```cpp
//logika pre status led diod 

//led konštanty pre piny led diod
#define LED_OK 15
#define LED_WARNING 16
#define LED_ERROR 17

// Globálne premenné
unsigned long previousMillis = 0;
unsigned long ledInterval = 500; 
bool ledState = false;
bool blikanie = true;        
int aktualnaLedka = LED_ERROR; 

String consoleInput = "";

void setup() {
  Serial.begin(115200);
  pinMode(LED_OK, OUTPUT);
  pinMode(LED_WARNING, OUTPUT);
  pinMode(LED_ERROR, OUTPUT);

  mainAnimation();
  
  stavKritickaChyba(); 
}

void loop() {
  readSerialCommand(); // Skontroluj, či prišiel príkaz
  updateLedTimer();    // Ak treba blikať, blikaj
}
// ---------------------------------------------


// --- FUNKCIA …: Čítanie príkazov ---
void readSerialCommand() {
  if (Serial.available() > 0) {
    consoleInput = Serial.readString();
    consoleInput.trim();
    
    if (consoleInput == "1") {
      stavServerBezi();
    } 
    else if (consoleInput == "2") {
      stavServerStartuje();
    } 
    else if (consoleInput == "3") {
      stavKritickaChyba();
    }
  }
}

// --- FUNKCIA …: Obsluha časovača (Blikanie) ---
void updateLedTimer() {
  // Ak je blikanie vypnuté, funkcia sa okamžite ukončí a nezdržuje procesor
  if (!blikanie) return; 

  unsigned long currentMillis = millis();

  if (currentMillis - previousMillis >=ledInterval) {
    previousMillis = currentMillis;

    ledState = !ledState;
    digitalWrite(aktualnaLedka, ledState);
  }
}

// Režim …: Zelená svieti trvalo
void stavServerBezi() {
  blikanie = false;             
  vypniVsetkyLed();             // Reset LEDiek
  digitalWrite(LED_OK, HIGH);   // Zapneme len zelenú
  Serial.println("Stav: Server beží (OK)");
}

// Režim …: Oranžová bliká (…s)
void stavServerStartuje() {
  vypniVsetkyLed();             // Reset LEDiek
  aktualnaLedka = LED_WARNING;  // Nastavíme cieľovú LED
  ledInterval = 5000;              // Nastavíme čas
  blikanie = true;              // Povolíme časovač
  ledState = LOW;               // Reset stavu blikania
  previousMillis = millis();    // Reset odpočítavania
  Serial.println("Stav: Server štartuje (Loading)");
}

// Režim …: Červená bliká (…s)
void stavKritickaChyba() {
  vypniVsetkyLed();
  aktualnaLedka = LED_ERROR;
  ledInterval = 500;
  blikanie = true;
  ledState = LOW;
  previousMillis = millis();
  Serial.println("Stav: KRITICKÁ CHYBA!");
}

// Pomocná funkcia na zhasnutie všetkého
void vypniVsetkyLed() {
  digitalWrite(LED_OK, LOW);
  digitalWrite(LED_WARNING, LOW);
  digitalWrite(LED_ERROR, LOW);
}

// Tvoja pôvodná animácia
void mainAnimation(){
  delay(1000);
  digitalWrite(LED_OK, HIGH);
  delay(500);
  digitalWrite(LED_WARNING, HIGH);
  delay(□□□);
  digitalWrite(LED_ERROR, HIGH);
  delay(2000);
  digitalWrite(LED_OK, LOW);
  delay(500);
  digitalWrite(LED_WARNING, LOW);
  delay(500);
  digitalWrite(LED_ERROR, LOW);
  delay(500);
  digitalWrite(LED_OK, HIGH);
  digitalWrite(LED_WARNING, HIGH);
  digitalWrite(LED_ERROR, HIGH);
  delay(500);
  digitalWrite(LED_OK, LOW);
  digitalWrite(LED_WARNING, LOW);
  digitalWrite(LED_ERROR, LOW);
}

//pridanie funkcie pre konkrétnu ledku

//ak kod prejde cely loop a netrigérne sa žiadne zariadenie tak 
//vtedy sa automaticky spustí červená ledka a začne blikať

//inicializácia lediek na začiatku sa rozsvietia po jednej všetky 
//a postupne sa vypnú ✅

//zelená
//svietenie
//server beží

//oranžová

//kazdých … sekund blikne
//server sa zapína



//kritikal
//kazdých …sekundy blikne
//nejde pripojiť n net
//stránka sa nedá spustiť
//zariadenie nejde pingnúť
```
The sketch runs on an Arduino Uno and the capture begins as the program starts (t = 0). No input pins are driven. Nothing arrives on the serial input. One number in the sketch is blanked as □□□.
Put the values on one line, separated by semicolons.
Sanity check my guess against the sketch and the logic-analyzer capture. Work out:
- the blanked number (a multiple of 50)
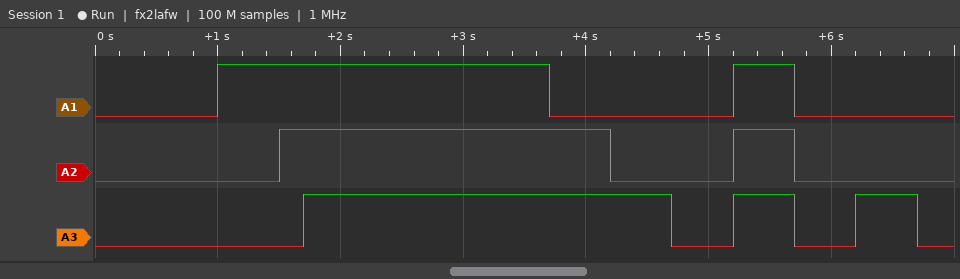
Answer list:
200
